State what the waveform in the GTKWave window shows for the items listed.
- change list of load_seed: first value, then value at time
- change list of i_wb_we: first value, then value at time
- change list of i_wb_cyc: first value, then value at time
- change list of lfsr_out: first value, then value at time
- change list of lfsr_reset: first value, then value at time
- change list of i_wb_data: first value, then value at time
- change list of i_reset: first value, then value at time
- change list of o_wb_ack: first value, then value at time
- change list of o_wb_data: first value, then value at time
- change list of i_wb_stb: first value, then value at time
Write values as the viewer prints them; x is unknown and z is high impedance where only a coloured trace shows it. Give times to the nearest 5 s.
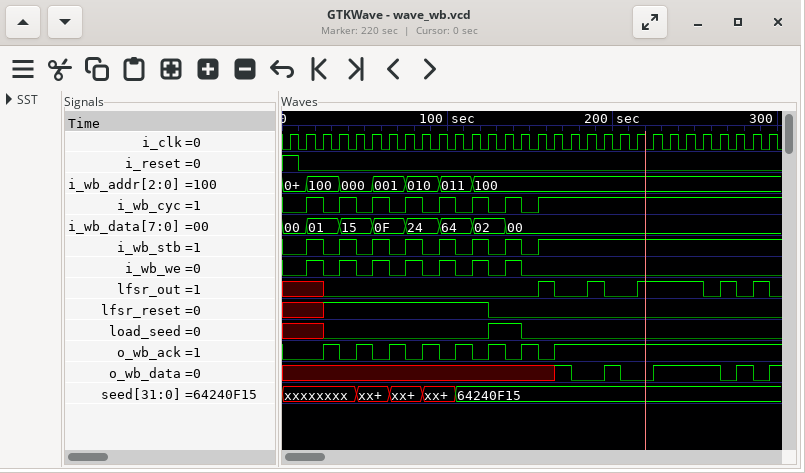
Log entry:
x, 0 at 25 s, 1 at 125 s, 0 at 145 s
0, 1 at 15 s, 0 at 25 s, 1 at 35 s, 0 at 45 s, 1 at 55 s, 0 at 65 s, 1 at 75 s, 0 at 85 s, 1 at 95 s, 0 at 105 s, 1 at 115 s, 0 at 125 s, 1 at 135 s, 0 at 145 s
0, 1 at 15 s, 0 at 25 s, 1 at 35 s, 0 at 45 s, 1 at 55 s, 0 at 65 s, 1 at 75 s, 0 at 85 s, 1 at 95 s, 0 at 105 s, 1 at 115 s, 0 at 125 s, 1 at 135 s, 0 at 145 s, 1 at 155 s
x, 0 at 25 s, 1 at 155 s, 0 at 165 s, 1 at 185 s, 0 at 195 s, 1 at 215 s, 0 at 255 s, 1 at 265 s, 0 at 275 s, 1 at 285 s, 0 at 295 s
x, 1 at 25 s, 0 at 125 s
00, 01 at 15 s, 15 at 35 s, 0F at 55 s, 24 at 75 s, 64 at 95 s, 02 at 115 s, 00 at 135 s
1, 0 at 10 s
0, 1 at 25 s, 0 at 35 s, 1 at 45 s, 0 at 55 s, 1 at 65 s, 0 at 75 s, 1 at 85 s, 0 at 95 s, 1 at 105 s, 0 at 115 s, 1 at 125 s, 0 at 135 s, 1 at 145 s, 0 at 155 s, 1 at 165 s
x, 1 at 165 s, 0 at 175 s, 1 at 195 s, 0 at 205 s, 1 at 225 s, 0 at 265 s, 1 at 275 s, 0 at 285 s, 1 at 295 s
0, 1 at 15 s, 0 at 25 s, 1 at 35 s, 0 at 45 s, 1 at 55 s, 0 at 65 s, 1 at 75 s, 0 at 85 s, 1 at 95 s, 0 at 105 s, 1 at 115 s, 0 at 125 s, 1 at 135 s, 0 at 145 s, 1 at 155 s
